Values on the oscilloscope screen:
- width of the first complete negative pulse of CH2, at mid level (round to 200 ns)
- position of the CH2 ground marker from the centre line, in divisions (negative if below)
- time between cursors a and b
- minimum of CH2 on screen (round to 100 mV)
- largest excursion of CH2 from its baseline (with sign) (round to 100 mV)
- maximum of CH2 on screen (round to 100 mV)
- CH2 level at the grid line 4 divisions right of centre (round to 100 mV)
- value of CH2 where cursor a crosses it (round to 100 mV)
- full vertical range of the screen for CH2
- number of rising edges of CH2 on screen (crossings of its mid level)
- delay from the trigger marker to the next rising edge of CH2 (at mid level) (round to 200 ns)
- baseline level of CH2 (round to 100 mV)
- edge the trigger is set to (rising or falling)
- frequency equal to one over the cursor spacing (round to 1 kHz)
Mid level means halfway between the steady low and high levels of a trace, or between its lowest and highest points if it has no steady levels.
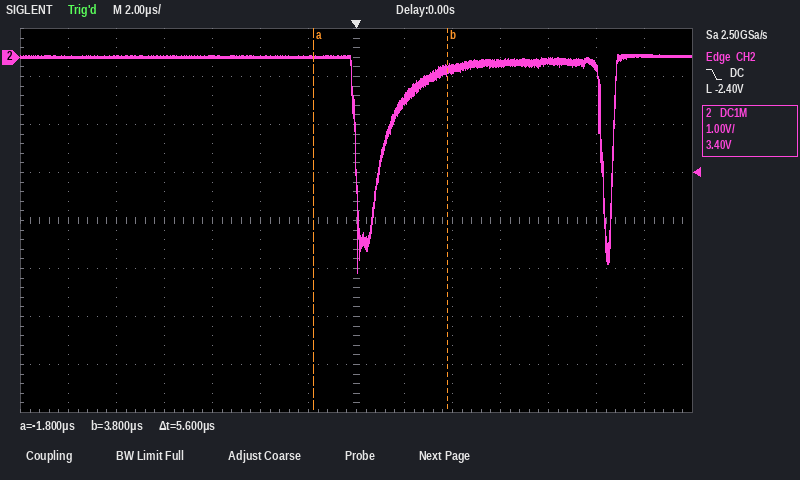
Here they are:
1.0 µs
+3.4 div
5.6 µs
-4.5 V
-4.5 V
100 mV
-100 mV
0.0 V
8 V
2
1.0 µs
0.0 V
falling
179 kHz
